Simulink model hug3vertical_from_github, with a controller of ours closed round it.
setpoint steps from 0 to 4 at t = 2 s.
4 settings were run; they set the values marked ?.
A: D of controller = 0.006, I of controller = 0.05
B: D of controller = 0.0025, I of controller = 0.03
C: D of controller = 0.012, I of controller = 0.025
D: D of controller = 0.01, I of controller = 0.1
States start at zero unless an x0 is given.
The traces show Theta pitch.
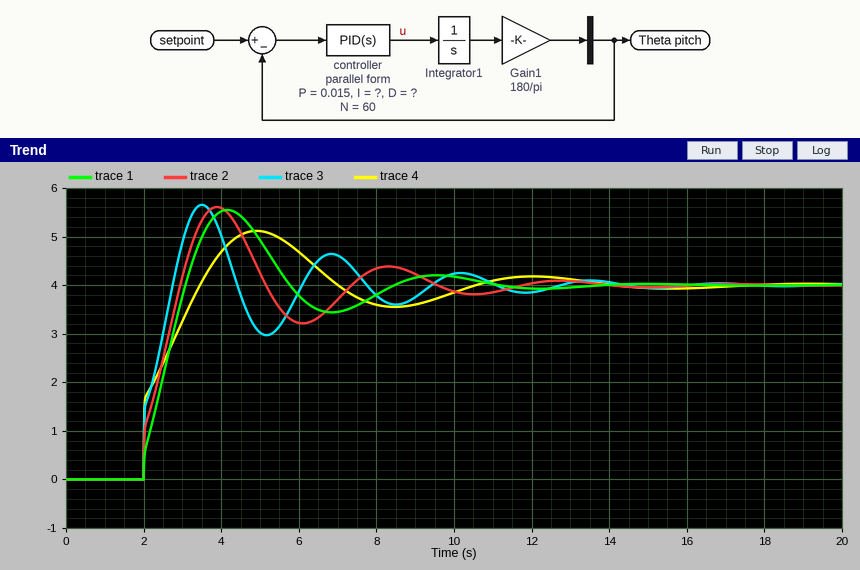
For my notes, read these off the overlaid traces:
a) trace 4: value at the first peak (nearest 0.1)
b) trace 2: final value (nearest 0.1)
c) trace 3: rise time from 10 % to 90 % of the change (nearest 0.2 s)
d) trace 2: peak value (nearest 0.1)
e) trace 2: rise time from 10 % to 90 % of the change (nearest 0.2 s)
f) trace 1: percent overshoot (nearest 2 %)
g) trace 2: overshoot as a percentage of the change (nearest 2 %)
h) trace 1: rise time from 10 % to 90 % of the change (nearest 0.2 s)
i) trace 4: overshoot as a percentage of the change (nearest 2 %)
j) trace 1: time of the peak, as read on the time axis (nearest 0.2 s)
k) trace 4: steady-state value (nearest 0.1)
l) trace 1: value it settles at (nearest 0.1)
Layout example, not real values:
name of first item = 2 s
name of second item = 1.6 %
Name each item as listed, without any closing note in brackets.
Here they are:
trace 4: value at the first peak = 5.1
trace 2: final value = 4.0
trace 3: rise time from 10 % to 90 % of the change = 0.6 s
trace 2: peak value = 5.6
trace 2: rise time from 10 % to 90 % of the change = 0.8 s
trace 1: percent overshoot = 38 %
trace 2: overshoot as a percentage of the change = 40 %
trace 1: rise time from 10 % to 90 % of the change = 1.0 s
trace 4: overshoot as a percentage of the change = 28 %
trace 1: time of the peak, as read on the time axis = 4.2 s
trace 4: steady-state value = 4.0
trace 1: value it settles at = 4.0
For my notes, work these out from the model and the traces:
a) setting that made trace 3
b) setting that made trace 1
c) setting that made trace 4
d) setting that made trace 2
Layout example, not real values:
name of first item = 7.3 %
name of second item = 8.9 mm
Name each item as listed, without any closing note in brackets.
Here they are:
setting that made trace 3 = D
setting that made trace 1 = B
setting that made trace 4 = C
setting that made trace 2 = A
